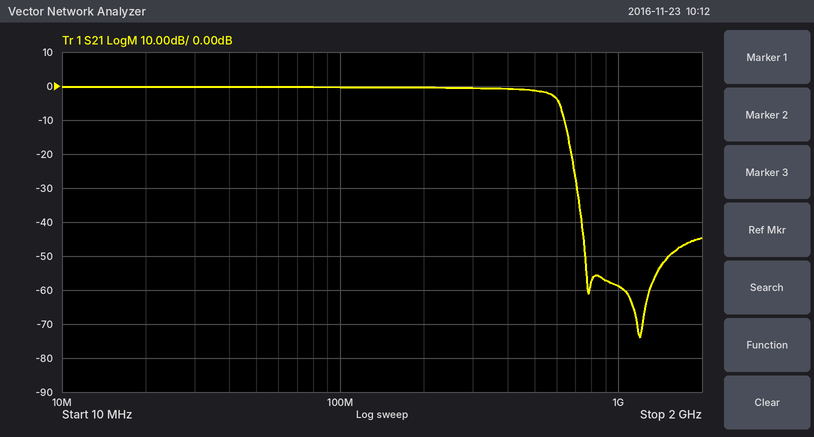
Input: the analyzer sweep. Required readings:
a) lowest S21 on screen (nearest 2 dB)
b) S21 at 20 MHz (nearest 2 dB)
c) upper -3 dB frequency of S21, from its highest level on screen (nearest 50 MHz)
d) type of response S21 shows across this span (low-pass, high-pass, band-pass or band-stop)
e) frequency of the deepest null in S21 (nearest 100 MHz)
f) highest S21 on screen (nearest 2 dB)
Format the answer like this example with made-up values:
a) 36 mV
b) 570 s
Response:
a) -74 dB
b) 0 dB
c) 600 MHz
d) low-pass
e) 1.2 GHz
f) 0 dB
